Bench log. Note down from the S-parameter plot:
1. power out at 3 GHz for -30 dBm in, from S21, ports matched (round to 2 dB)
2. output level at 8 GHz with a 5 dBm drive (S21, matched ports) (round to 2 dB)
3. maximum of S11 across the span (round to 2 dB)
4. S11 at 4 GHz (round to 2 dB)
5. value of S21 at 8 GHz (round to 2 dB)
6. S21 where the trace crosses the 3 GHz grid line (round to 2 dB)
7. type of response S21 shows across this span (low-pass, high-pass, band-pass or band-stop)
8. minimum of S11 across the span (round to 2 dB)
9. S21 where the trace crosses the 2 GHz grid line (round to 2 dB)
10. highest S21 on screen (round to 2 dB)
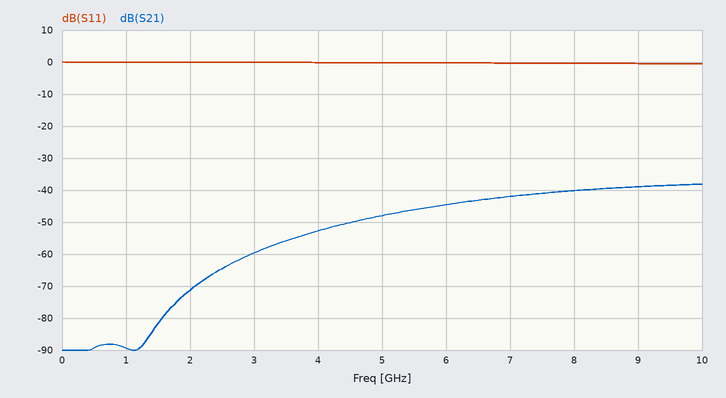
-90 dBm
-36 dBm
0 dB
0 dB
-40 dB
-60 dB
high-pass
0 dB
-72 dB
-38 dB
